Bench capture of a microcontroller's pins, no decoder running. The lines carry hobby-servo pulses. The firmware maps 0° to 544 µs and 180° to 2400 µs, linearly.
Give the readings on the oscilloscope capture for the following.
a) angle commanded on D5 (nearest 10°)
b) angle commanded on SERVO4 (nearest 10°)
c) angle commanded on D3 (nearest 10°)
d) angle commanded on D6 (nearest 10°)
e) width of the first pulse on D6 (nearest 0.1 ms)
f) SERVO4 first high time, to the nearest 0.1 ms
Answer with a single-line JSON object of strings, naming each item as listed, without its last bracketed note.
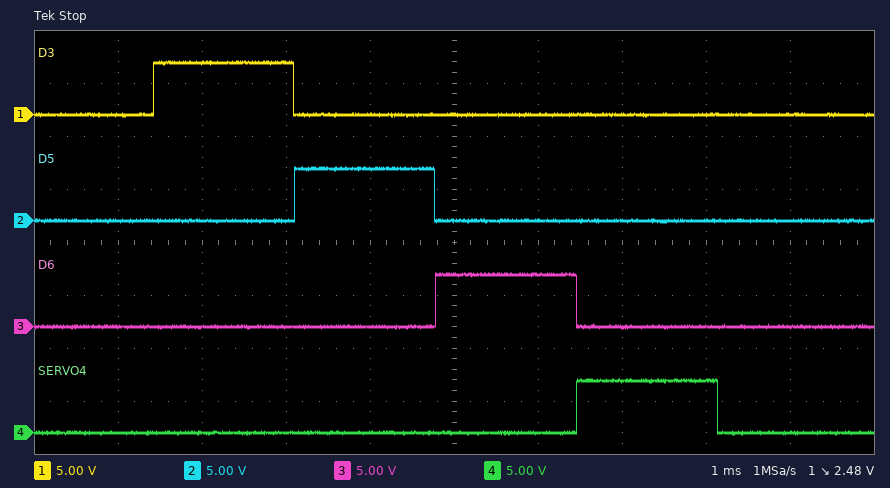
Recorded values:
{"angle commanded on D5": "110°", "angle commanded on SERVO4": "110°", "angle commanded on D3": "110°", "angle commanded on D6": "110°", "width of the first pulse on D6": "1.7 ms", "SERVO4 first high time, to the nearest 0.1 ms": "1.7 ms"}
